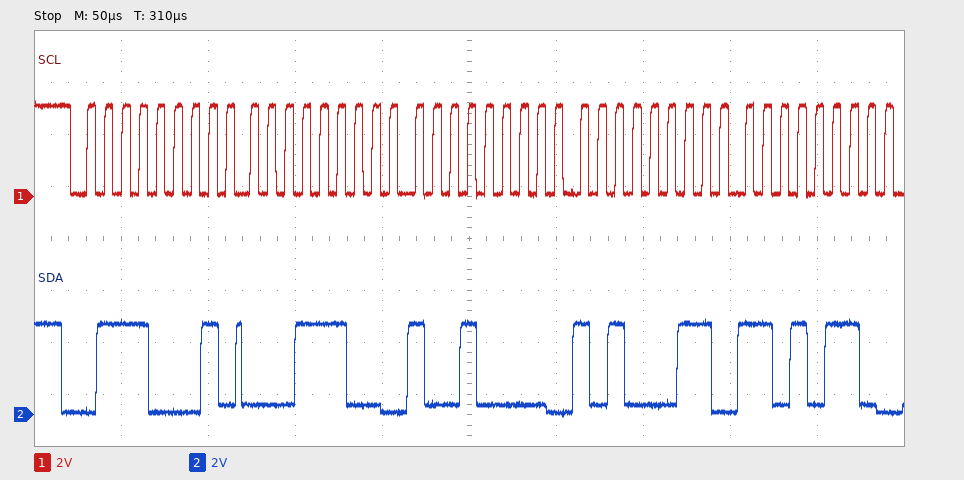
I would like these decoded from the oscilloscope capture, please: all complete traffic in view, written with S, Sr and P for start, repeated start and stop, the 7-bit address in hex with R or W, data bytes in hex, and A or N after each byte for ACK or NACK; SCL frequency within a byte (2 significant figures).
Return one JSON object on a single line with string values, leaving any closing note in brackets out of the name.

{"all complete traffic in view, written with S, Sr and P for start, repeated start and stop, the 7-bit address in hex with R or W, data bytes in hex, and A or N after each byte for ACK or NACK": "S 38R A 1C A 90 A A3 A D6 A", "SCL frequency within a byte": "100 kHz"}
